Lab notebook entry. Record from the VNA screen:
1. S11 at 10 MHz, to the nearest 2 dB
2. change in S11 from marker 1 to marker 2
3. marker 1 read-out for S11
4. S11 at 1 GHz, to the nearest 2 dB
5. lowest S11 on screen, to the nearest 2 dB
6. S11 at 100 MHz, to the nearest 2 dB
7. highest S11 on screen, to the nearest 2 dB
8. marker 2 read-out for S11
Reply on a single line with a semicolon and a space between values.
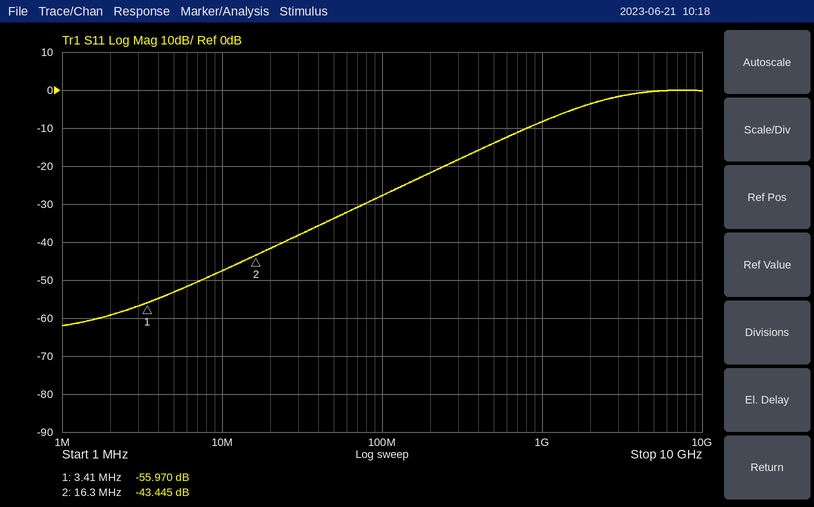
-48 dB; 12.525 dB; -55.970 dB; -8 dB; -62 dB; -28 dB; 0 dB; -43.445 dB
